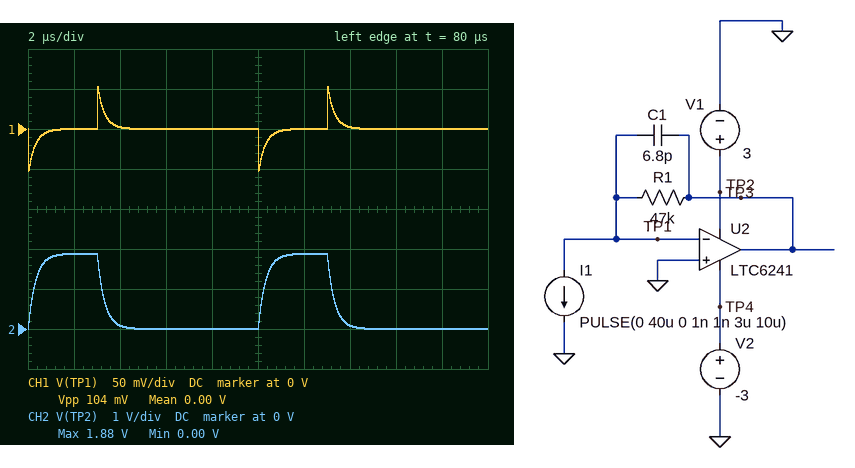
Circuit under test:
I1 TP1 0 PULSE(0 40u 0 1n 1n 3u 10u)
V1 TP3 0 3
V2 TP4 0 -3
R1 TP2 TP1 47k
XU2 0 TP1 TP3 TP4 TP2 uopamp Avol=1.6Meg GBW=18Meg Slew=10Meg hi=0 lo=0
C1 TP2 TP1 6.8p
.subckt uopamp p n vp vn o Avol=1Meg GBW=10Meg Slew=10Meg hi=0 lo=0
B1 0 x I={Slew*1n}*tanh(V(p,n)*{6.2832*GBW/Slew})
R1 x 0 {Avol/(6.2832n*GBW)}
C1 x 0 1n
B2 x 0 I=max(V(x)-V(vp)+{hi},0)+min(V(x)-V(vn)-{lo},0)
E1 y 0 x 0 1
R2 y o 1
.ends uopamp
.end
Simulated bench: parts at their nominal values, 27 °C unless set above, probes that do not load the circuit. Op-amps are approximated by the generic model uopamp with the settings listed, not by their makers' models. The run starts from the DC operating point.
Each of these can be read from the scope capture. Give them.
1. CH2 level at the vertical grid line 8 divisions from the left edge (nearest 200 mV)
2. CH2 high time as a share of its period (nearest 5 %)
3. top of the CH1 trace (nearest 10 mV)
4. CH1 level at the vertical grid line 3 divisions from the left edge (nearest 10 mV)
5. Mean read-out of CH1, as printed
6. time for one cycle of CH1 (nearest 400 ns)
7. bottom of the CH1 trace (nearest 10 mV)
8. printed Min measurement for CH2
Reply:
0 V
30 %
50 mV
0 V
0.00 V
10.0 µs
-50 mV
0.00 V
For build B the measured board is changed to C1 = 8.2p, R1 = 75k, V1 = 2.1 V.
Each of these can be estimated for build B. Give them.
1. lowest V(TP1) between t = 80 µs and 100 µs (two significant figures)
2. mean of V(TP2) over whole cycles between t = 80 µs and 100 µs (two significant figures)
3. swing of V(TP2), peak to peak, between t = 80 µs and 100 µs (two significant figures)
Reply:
-870 mV
740 mV
2.1 V
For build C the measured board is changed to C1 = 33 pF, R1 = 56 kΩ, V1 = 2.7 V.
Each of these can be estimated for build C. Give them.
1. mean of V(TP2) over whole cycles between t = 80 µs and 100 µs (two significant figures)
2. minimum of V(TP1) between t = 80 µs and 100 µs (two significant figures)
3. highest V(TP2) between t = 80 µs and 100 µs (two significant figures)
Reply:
670 mV
-10 mV
1.8 V
